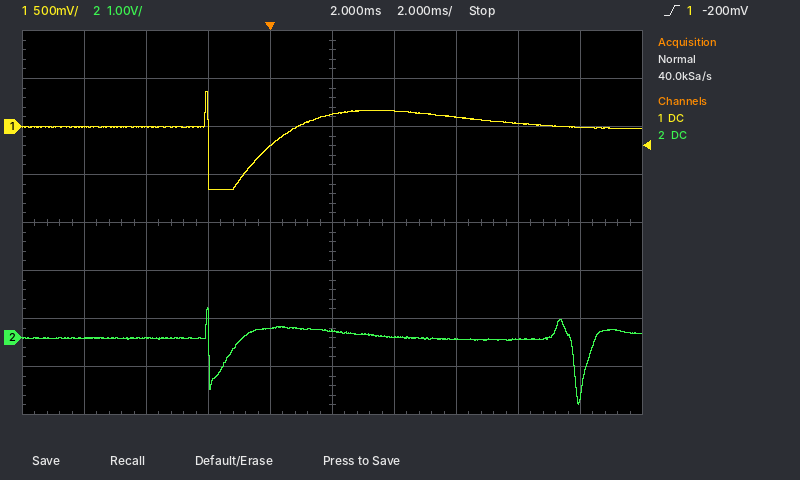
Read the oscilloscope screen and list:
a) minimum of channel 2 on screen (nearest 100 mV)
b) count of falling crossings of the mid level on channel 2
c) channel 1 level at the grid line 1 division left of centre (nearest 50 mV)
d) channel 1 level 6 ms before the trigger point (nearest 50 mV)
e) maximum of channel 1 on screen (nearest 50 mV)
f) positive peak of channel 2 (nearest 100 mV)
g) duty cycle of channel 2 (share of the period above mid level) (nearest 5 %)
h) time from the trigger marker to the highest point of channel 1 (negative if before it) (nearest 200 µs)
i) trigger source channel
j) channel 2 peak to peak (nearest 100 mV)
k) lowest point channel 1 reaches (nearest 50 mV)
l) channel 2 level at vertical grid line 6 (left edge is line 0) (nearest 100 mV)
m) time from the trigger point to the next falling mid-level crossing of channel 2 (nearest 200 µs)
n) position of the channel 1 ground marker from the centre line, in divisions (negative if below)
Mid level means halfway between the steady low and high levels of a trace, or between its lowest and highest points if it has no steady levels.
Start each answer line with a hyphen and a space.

- -1.4 V
- 2
- -200 mV
- 0 mV
- 350 mV
- 600 mV
- 95 %
- -2.0 ms
- channel 1
- 2.0 V
- -650 mV
- 0.0 V
- 9.8 ms
- +2.0 div
